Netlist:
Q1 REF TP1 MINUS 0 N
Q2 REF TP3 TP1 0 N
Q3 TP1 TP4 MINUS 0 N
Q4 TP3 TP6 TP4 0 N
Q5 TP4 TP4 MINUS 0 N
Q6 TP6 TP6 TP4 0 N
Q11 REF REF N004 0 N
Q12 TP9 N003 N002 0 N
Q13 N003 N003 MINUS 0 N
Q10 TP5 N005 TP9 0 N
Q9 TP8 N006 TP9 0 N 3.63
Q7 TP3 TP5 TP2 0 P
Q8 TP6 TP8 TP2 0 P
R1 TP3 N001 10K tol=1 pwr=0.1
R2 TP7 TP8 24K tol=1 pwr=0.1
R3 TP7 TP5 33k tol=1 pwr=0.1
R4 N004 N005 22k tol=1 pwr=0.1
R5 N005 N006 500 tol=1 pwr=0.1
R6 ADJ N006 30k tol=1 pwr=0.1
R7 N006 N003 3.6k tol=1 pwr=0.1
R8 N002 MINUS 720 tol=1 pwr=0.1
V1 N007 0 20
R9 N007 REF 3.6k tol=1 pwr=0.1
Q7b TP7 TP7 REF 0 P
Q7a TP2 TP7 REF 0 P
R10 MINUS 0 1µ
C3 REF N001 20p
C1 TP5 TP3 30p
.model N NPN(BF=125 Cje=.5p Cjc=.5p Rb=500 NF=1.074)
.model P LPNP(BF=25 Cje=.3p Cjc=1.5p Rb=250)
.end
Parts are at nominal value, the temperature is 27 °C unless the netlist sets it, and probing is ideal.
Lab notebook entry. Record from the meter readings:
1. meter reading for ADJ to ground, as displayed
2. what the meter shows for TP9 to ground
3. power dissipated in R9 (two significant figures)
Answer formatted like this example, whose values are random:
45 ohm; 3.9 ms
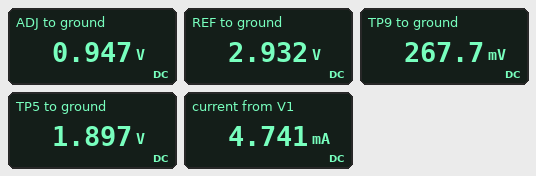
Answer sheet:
0.947 V; 267.7 mV; 81 mW
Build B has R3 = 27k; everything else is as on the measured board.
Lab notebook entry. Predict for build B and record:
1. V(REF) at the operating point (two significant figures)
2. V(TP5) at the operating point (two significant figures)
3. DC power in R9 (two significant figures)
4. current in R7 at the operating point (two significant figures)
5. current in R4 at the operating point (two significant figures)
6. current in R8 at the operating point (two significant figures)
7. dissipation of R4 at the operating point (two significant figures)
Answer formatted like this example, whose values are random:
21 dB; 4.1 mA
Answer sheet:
3.2 V; 2.2 V; 78 mW; 65 µA; 66 µA; 30 µA; 95 µW
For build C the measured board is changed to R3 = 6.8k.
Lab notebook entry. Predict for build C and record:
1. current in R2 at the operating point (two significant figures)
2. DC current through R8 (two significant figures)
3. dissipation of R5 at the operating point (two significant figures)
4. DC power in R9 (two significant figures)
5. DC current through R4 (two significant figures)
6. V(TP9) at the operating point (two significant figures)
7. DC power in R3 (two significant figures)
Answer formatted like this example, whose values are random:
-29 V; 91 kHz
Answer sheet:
9.3 µA; 44 µA; 9.7 µW; 61 mW; 140 µA; 610 mV; 7.4 µW
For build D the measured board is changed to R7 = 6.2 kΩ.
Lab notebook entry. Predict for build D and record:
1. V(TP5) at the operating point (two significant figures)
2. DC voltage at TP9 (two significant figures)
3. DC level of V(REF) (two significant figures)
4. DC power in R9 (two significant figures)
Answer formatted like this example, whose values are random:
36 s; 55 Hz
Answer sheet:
2.0 V; 410 mV; 3.1 V; 80 mW
